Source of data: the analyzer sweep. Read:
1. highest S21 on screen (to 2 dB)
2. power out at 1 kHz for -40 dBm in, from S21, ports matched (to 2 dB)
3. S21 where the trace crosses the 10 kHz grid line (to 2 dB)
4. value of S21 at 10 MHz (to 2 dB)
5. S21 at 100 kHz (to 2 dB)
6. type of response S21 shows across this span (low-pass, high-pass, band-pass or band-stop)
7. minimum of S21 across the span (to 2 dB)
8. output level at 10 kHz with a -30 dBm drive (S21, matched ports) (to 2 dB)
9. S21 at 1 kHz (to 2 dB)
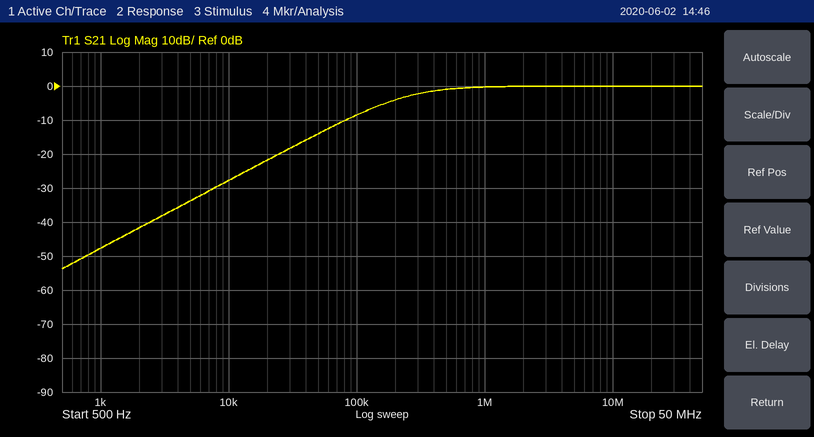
0 dB
-88 dBm
-28 dB
0 dB
-8 dB
high-pass
-54 dB
-58 dBm
-48 dB
